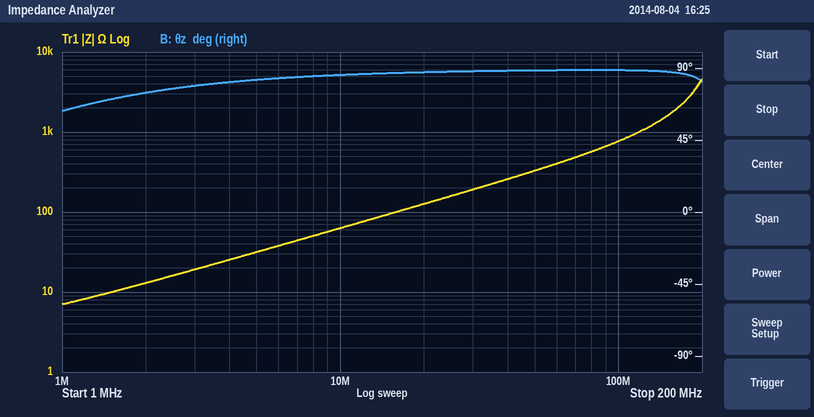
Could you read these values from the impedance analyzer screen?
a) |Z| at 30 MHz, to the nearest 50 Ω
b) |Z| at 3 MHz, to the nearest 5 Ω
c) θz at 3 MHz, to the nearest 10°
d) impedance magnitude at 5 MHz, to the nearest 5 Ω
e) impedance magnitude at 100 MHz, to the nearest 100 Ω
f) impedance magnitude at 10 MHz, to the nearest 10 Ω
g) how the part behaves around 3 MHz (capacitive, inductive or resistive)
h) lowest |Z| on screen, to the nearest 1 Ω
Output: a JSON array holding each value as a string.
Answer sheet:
["200 Ω", "20 Ω", "80°", "30 Ω", "800 Ω", "60 Ω", "inductive", "7 Ω"]
